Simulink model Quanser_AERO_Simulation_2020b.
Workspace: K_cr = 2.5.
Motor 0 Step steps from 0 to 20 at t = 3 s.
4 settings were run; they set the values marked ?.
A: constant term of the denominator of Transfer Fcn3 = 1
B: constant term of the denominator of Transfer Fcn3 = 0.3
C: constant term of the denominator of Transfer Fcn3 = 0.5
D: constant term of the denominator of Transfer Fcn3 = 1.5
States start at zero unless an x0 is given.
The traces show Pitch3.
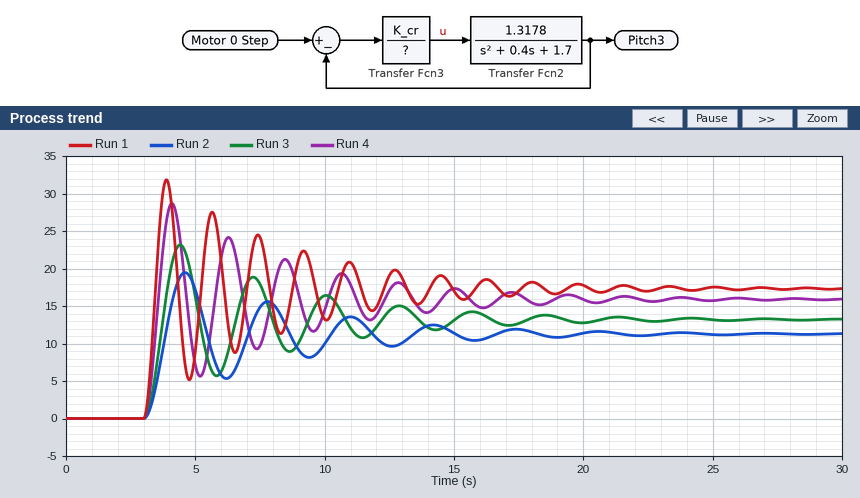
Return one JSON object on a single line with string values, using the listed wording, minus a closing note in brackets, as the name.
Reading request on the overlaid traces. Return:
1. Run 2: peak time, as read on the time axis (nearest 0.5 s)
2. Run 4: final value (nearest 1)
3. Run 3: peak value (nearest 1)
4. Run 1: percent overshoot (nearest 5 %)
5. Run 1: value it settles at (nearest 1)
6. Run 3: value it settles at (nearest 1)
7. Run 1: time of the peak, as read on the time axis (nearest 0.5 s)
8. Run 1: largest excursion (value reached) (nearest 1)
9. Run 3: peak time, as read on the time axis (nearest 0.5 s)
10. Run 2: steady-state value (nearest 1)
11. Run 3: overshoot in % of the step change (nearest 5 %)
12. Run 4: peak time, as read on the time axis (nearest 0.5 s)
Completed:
{"Run 2: peak time, as read on the time axis": "4.5 s", "Run 4: final value": "16", "Run 3: peak value": "23", "Run 1: percent overshoot": "85 %", "Run 1: value it settles at": "17", "Run 3: value it settles at": "13", "Run 1: time of the peak, as read on the time axis": "4.0 s", "Run 1: largest excursion (value reached)": "32", "Run 3: peak time, as read on the time axis": "4.5 s", "Run 2: steady-state value": "11", "Run 3: overshoot in % of the step change": "75 %", "Run 4: peak time, as read on the time axis": "4.0 s"}
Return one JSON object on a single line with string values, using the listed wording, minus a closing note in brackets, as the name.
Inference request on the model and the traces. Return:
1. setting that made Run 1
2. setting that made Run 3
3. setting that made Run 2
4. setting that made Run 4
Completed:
{"setting that made Run 1": "B", "setting that made Run 3": "A", "setting that made Run 2": "D", "setting that made Run 4": "C"}
